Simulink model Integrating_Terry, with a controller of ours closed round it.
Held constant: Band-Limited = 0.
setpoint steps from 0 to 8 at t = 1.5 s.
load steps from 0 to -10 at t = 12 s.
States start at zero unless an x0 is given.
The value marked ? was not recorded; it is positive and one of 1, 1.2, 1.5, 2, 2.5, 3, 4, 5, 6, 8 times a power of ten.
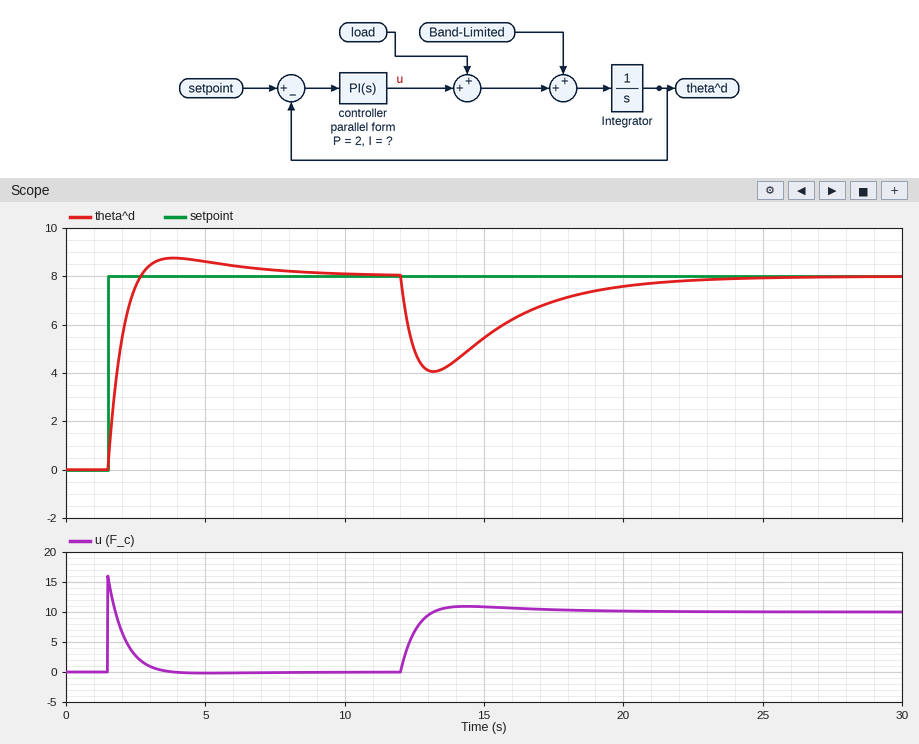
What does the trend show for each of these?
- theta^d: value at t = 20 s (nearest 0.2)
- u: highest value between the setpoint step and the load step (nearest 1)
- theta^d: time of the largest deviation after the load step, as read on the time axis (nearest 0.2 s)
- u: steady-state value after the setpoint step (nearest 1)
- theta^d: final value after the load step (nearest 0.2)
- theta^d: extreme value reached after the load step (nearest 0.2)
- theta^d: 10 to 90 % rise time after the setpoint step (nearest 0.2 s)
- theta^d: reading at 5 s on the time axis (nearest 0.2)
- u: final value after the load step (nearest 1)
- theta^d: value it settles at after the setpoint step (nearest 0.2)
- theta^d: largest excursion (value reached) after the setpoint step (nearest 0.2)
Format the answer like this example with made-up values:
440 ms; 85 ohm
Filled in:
7.6; 16; 13.2 s; 0; 8.0; 4.0; 0.8 s; 8.6; 10; 8.0; 8.8
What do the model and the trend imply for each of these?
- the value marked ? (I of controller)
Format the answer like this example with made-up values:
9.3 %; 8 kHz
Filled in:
0.6
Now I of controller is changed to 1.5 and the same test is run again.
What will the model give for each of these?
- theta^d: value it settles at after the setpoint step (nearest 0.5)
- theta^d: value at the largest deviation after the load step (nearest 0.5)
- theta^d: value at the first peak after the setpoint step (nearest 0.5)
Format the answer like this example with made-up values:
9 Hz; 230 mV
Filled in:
8.0; 4.5; 9.5
